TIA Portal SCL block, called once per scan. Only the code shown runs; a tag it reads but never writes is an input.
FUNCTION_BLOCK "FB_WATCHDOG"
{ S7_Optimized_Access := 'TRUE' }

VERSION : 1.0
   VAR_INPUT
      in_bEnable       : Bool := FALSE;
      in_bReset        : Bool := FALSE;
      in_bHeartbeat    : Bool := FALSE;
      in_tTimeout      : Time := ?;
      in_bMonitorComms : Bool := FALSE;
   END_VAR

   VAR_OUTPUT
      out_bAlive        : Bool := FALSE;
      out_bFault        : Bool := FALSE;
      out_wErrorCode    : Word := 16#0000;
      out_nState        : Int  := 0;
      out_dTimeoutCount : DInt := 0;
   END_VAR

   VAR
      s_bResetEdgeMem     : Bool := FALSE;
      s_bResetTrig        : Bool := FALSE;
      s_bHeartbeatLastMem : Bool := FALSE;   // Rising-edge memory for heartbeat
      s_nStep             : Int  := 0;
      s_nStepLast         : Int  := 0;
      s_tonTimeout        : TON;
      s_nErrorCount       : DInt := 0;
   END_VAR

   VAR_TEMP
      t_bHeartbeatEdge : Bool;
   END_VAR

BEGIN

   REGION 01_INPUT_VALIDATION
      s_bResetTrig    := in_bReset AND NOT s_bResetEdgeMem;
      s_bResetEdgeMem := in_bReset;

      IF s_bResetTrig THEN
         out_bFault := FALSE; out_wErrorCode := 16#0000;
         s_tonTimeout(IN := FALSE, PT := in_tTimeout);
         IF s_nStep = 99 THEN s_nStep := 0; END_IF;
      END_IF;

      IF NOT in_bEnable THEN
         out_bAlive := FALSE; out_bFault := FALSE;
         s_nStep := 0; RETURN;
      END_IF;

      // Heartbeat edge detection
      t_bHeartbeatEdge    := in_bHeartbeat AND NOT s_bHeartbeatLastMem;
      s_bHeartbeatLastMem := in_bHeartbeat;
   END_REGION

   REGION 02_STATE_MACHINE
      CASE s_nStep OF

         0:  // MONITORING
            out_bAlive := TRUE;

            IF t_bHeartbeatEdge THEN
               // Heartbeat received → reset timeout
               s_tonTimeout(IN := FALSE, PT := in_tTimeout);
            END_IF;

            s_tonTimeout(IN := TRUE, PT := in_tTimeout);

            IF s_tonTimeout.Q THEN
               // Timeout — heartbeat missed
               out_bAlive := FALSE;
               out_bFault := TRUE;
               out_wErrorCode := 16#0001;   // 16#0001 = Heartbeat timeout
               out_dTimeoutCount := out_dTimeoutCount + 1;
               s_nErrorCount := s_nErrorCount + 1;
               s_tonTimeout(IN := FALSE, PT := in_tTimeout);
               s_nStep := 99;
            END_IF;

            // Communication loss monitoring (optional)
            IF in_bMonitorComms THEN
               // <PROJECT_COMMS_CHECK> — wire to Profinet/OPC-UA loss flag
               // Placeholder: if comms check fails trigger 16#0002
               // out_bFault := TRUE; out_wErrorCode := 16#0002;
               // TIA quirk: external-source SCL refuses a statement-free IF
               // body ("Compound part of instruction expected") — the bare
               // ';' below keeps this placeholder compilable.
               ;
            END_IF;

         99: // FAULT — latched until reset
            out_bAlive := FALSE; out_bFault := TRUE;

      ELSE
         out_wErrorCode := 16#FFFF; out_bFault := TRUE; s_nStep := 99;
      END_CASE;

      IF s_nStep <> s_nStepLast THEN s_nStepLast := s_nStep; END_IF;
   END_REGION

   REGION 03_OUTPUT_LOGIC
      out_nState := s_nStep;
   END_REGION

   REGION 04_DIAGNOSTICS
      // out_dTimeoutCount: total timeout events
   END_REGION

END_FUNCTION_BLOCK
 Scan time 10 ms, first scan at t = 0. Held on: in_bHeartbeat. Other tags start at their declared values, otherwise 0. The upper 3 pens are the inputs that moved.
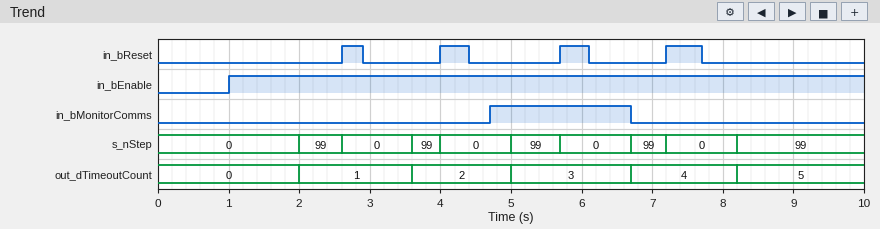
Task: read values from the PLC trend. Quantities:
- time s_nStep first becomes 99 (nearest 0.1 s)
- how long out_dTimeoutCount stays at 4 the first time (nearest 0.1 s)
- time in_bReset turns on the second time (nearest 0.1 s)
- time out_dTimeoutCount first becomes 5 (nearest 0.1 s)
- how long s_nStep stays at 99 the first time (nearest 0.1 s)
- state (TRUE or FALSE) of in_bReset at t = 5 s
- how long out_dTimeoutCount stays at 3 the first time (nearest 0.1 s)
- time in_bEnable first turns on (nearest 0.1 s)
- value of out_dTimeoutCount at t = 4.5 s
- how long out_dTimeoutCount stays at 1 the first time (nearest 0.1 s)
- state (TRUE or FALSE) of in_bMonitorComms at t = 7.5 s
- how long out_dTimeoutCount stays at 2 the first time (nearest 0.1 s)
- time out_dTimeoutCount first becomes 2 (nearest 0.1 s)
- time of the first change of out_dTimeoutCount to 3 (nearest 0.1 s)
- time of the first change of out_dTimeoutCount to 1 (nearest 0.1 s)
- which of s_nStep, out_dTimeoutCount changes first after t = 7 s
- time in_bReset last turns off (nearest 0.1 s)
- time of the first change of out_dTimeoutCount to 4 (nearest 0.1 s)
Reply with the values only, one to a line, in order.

2.0 s
1.5 s
4.0 s
8.2 s
0.6 s
FALSE
1.7 s
1.0 s
2
1.6 s
FALSE
1.4 s
3.6 s
5.0 s
2.0 s
s_nStep
7.7 s
6.7 s
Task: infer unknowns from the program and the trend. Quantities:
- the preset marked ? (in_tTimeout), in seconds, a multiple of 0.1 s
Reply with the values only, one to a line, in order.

1.0 s
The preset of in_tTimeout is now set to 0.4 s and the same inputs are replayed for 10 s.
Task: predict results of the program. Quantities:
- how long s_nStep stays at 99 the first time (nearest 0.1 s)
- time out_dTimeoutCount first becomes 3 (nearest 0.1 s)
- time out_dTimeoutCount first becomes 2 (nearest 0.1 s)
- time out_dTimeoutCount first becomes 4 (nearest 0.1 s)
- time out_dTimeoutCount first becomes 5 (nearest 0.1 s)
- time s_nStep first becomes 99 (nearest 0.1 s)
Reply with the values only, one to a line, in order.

1.2 s
4.4 s
3.0 s
6.1 s
7.6 s
1.4 s
